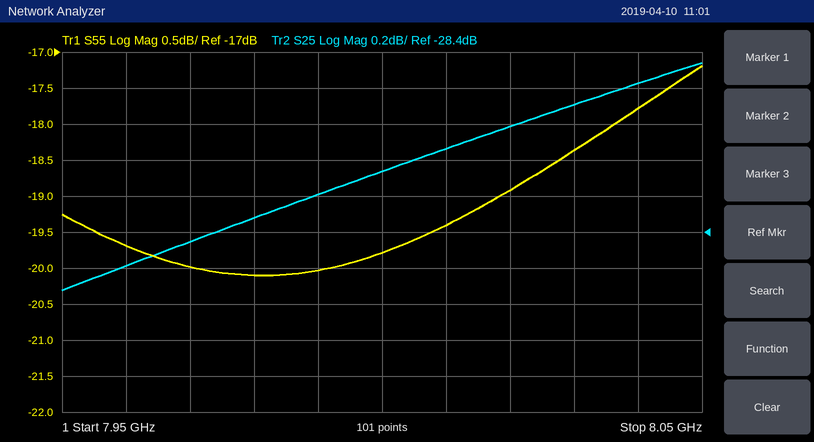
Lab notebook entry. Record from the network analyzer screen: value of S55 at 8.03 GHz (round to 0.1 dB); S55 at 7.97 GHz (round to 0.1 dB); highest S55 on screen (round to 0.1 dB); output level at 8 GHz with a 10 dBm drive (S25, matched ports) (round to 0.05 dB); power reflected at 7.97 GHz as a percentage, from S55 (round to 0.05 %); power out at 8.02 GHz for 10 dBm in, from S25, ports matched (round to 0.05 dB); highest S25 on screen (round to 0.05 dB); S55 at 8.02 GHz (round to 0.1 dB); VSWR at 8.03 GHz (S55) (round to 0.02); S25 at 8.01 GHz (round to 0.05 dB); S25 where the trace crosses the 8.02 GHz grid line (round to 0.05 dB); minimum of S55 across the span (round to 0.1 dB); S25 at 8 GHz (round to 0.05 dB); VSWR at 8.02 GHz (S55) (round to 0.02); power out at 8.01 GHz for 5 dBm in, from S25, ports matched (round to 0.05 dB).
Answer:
-18.4 dB
-20.0 dB
-17.2 dB
-18.05 dBm
1.00 %
-17.80 dBm
-27.45 dB
-18.9 dB
1.28
-27.95 dB
-27.80 dB
-20.1 dB
-28.05 dB
1.26
-22.95 dBm
